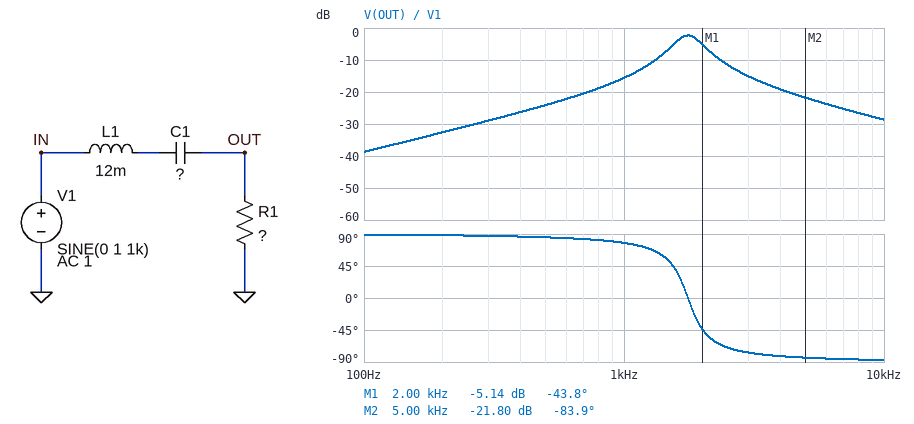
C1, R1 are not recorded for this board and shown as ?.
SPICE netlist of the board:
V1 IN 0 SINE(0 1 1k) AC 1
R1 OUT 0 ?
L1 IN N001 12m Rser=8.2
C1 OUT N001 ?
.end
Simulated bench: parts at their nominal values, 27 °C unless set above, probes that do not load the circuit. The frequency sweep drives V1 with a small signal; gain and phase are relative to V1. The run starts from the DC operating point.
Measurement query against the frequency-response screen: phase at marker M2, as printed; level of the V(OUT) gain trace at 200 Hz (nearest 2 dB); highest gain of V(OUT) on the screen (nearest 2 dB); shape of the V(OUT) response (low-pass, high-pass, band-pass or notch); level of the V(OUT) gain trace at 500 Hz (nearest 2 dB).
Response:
-83.9 deg
-32 dB
-2 dB
band-pass
-24 dB
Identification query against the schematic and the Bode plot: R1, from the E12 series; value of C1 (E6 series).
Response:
27 Ω
680 nF
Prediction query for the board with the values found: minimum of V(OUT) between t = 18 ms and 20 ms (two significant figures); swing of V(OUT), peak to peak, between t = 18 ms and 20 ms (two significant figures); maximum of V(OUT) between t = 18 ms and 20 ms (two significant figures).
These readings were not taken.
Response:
-170 mV
330 mV
170 mV
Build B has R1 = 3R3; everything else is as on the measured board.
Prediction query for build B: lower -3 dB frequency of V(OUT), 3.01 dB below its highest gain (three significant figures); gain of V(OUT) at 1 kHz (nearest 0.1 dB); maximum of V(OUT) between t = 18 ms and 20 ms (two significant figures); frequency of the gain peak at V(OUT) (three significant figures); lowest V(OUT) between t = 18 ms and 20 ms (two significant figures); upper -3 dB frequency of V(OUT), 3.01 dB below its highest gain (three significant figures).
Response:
1.69 kHz
-33.7 dB
21 mV
1.76 kHz
-21 mV
1.84 kHz
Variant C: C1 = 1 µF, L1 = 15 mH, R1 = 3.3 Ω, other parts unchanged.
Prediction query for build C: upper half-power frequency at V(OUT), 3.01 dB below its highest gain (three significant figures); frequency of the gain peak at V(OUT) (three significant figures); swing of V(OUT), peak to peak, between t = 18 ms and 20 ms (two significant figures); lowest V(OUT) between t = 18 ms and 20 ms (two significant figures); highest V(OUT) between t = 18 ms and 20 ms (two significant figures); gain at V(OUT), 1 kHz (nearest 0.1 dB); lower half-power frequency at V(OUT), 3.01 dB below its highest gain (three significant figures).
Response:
1.36 kHz
1.30 kHz
100 mV
-50 mV
50 mV
-26.0 dB
1.24 kHz
